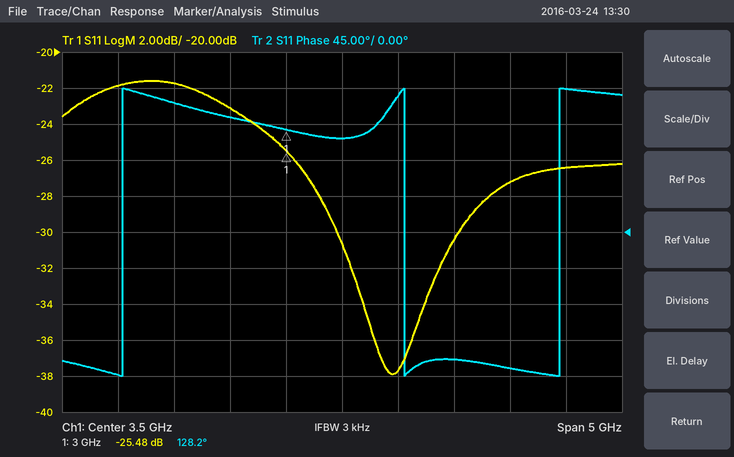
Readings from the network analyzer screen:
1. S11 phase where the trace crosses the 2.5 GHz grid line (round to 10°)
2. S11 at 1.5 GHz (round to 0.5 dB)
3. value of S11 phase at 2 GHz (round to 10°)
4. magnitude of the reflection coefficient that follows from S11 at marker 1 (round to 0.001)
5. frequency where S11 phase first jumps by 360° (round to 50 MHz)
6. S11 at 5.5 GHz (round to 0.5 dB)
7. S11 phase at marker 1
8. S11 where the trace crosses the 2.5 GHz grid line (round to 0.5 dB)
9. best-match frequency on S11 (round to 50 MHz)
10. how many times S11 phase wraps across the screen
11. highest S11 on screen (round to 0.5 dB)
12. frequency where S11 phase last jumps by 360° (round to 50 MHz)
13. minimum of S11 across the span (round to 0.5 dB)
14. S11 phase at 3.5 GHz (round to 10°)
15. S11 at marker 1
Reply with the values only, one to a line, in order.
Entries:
140°
-22.0 dB
160°
0.053
1.55 GHz
-26.5 dB
128.2°
-23.0 dB
3.95 GHz
3
-21.5 dB
5.45 GHz
-38.0 dB
120°
-25.48 dB
